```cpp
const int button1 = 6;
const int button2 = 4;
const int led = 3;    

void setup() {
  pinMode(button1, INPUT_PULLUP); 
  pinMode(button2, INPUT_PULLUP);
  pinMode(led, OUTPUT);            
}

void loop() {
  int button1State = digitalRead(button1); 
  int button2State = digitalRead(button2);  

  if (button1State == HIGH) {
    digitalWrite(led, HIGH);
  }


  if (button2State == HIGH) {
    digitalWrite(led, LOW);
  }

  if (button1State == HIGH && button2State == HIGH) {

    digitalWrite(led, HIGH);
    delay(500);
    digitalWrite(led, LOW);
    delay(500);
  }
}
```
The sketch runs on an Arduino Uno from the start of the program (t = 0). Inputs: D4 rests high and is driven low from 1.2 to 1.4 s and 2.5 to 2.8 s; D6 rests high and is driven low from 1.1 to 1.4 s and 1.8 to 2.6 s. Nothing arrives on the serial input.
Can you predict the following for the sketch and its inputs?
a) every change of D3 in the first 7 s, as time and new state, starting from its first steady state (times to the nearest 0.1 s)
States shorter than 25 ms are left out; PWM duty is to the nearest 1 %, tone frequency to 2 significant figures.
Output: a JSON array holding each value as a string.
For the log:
["0 s high; 0.5 s low; 1 s high; 1.5 s low; 2.6 s high; 3.3 s low; 3.8 s high; 4.3 s low; 4.8 s high; 5.3 s low; 5.8 s high; 6.3 s low; 6.8 s high"]
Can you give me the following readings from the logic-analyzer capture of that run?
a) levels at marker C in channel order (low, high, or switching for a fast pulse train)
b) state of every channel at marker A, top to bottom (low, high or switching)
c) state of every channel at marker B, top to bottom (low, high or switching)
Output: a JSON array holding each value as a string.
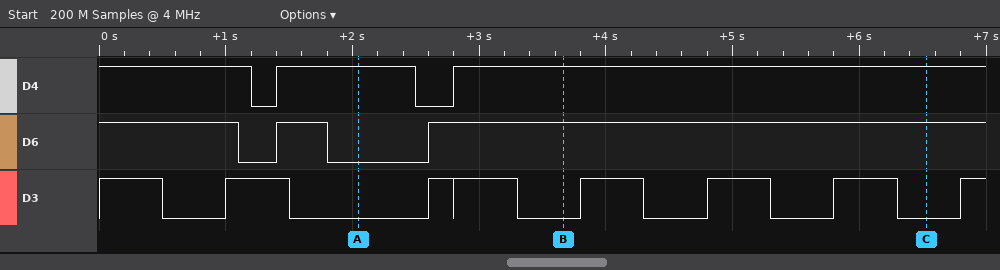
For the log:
["D4 high, D6 high, D3 low", "D4 high, D6 low, D3 low", "D4 high, D6 high, D3 low"]
